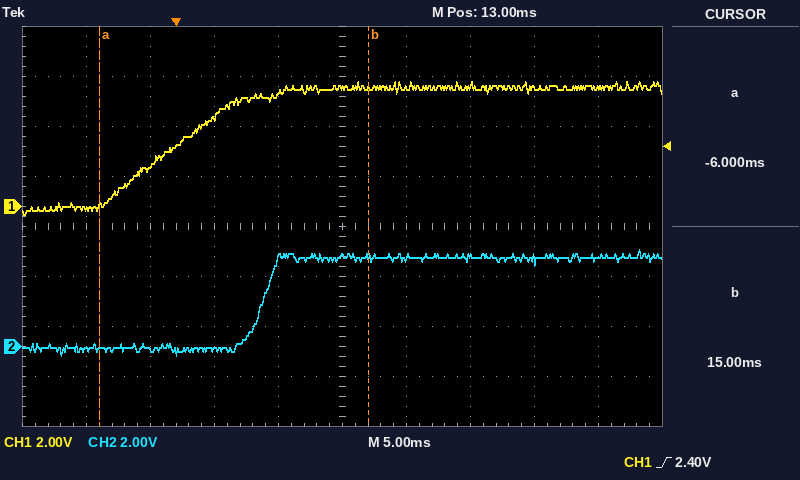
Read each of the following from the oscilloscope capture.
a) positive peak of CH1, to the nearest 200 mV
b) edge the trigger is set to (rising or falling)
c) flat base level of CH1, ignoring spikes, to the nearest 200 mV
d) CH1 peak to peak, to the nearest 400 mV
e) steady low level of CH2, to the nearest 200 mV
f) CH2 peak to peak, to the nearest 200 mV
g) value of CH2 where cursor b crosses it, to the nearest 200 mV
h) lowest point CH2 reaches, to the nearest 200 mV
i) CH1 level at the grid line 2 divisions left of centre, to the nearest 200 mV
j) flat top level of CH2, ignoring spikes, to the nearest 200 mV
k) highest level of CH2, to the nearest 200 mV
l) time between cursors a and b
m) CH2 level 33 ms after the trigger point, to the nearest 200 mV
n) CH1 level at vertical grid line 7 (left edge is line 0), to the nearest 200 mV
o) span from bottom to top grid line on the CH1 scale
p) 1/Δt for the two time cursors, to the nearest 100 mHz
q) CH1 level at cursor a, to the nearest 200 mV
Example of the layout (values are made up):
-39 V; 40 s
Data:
5.0 V; rising; 0.0 V; 5.2 V; 0.0 V; 4.2 V; 3.6 V; -400 mV; 3.6 V; 3.6 V; 3.8 V; 21.0 ms; 3.6 V; 4.8 V; 16 V; 47.6 Hz; 0.0 V
